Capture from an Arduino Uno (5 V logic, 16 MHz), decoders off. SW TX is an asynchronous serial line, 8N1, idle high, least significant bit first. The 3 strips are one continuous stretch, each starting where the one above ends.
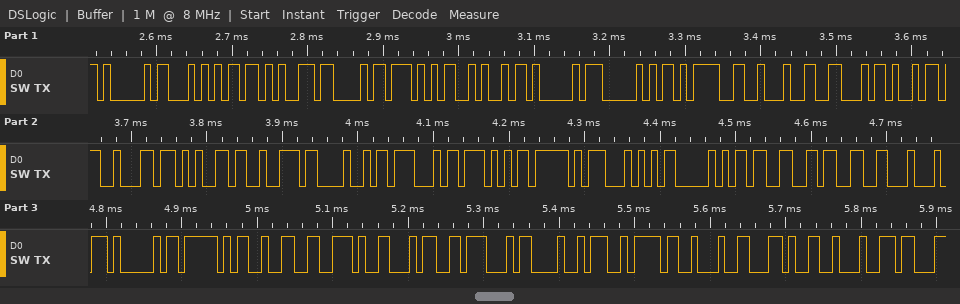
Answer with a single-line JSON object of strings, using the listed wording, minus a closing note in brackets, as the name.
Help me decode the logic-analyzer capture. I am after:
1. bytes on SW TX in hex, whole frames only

{"bytes on SW TX in hex, whole frames only": "41 54 2B 43 57 4A 41 50 3D 22 46 69 62 65 72 48 47 57 5F 54 50 33 33 44 41 5F 32 2E 34 47 48 7A 22 2C 22"}
